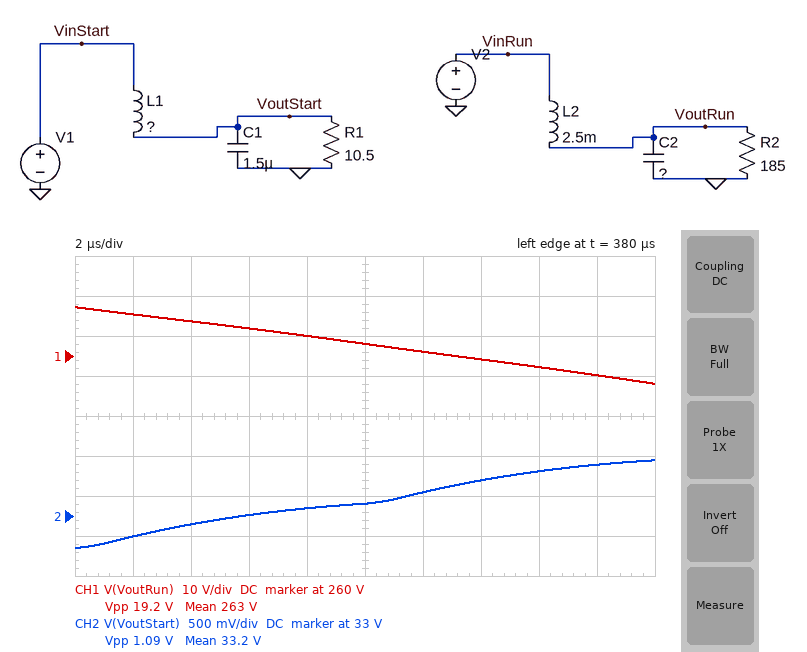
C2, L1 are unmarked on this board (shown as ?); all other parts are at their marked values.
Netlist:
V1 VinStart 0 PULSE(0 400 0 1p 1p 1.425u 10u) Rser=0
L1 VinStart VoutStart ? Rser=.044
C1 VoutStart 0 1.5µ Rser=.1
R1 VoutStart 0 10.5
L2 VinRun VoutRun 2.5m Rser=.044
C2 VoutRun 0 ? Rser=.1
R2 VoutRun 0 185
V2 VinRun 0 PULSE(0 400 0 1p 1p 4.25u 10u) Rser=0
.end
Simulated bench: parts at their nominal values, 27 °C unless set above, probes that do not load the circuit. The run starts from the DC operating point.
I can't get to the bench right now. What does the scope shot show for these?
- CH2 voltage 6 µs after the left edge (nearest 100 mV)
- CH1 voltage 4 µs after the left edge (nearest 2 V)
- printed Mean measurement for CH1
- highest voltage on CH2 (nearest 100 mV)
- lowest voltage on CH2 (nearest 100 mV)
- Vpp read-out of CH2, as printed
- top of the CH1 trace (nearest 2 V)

33.0 V
268 V
263 V
33.7 V
32.6 V
1.09 V
272 V
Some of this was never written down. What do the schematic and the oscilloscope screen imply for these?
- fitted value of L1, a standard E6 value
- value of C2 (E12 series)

4.7 mH
3.9 µF
